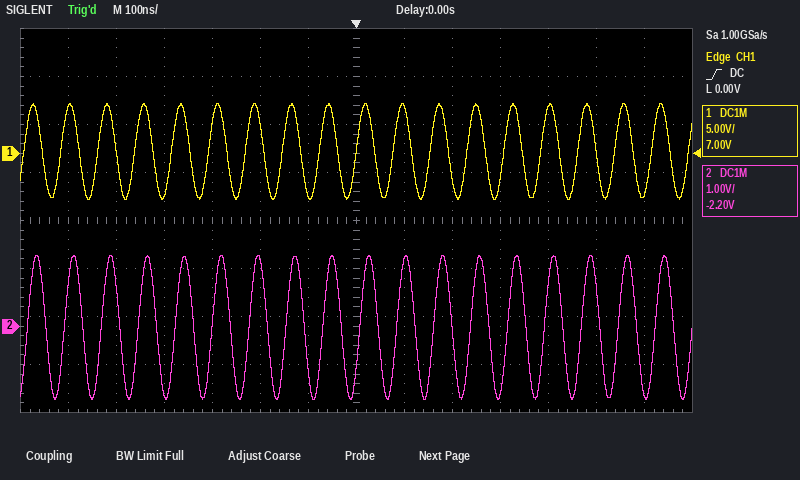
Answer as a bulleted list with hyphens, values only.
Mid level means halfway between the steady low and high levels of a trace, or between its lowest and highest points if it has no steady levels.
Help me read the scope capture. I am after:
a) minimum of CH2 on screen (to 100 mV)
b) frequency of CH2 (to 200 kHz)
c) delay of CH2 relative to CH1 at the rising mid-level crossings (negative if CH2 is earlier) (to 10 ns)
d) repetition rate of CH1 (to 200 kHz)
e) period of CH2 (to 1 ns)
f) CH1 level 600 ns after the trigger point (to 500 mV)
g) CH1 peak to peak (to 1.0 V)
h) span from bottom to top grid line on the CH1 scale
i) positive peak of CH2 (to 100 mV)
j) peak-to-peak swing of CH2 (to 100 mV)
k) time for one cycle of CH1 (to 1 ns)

- -1.5 V
- 13.0 MHz
- +10 ns
- 13.0 MHz
- 77 ns
- -4.0 V
- 10.0 V
- 40 V
- 1.5 V
- 3.0 V
- 77 ns
